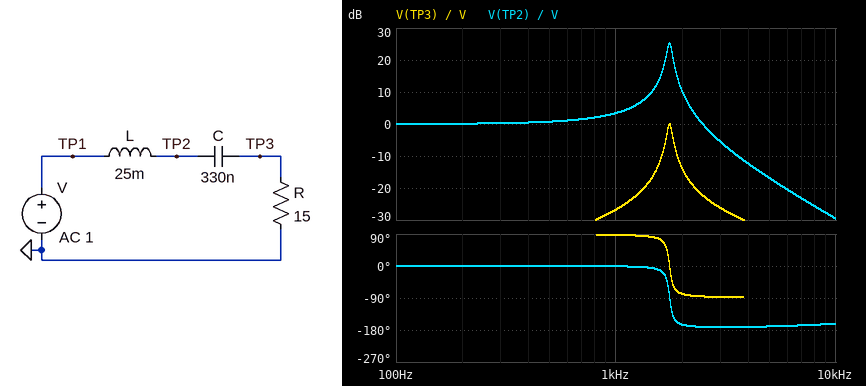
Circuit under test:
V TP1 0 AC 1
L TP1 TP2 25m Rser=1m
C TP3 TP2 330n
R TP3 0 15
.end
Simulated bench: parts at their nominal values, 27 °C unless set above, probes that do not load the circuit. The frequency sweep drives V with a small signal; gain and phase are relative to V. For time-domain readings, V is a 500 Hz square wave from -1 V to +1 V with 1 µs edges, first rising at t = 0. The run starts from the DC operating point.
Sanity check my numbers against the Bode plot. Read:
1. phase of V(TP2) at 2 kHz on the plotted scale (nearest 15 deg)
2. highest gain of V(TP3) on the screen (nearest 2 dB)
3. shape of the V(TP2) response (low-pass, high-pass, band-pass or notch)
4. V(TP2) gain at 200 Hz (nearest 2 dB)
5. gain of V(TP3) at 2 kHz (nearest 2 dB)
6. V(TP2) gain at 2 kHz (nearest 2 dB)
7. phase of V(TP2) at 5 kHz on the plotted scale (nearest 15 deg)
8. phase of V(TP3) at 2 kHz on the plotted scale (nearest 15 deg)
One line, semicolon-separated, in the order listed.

-165 deg; 0 dB; band-pass; 0 dB; -14 dB; 10 dB; -165 deg; -75 deg
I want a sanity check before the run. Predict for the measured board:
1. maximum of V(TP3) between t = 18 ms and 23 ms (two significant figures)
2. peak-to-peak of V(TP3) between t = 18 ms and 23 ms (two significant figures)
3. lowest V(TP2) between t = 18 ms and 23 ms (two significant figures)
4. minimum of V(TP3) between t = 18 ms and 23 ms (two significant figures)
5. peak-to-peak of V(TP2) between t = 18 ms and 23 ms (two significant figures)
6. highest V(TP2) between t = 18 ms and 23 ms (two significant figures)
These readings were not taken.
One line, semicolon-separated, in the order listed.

85 mV; 170 mV; -2.5 V; -85 mV; 5.0 V; 2.5 V
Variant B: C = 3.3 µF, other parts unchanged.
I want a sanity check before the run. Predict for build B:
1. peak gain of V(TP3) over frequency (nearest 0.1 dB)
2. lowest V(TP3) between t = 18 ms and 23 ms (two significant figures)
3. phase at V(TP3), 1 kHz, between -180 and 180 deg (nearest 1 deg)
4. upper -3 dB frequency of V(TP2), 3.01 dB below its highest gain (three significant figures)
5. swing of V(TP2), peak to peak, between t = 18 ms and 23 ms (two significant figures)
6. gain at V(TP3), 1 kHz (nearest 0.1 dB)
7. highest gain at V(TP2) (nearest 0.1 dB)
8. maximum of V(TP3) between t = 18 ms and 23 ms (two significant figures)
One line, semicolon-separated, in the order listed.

0 dB; -840 mV; -82 deg; 596 Hz; 11 V; -17.3 dB; 15.4 dB; 840 mV
